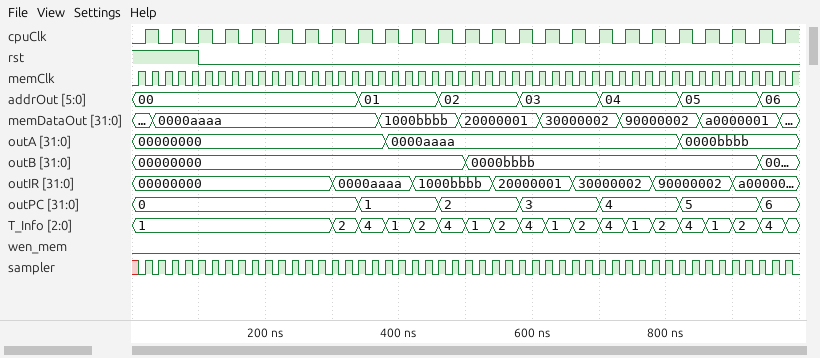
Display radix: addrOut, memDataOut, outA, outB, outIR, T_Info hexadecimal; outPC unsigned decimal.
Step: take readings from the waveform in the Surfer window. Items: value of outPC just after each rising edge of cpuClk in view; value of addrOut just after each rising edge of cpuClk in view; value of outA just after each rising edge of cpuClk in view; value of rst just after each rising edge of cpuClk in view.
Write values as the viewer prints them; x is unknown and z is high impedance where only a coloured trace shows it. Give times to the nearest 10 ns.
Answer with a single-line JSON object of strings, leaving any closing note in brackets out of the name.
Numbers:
{"value of outPC just after each rising edge of cpuClk in view": "0, 0, 0, 0, 0, 0, 0, 0, 1, 1, 1, 2, 2, 2, 3, 3, 3, 4, 4, 4, 5, 5, 5, 6, 6", "value of addrOut just after each rising edge of cpuClk in view": "00, 00, 00, 00, 00, 00, 00, 00, 01, 01, 01, 02, 02, 02, 03, 03, 03, 04, 04, 04, 05, 05, 05, 06, 06", "value of outA just after each rising edge of cpuClk in view": "00000000, 00000000, 00000000, 00000000, 00000000, 00000000, 00000000, 00000000, 00000000, 0000aaaa, 0000aaaa, 0000aaaa, 0000aaaa, 0000aaaa, 0000aaaa, 0000aaaa, 0000aaaa, 0000aaaa, 0000aaaa, 0000aaaa, 0000bbbb, 0000bbbb, 0000bbbb, 0000bbbb, 0000bbbb", "value of rst just after each rising edge of cpuClk in view": "1 1 0 0 0 0 0 0 0 0 0 0 0 0 0 0 0 0 0 0 0 0 0 0 0"}
